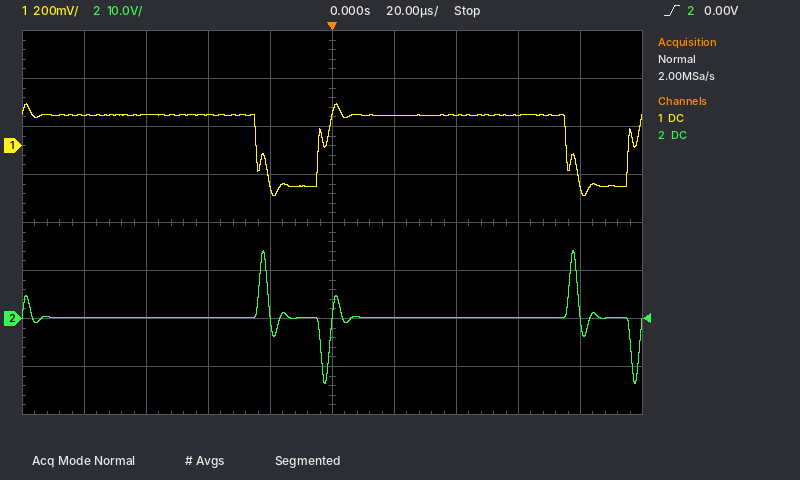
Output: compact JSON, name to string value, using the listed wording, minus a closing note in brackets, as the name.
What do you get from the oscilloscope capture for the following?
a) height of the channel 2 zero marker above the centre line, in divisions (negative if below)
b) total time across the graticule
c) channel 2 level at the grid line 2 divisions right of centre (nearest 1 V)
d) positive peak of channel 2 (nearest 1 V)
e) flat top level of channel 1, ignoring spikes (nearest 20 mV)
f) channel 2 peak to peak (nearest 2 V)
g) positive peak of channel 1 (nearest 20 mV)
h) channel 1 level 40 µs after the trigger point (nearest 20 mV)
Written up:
{"height of the channel 2 zero marker above the centre line, in divisions": "-2.0 div", "total time across the graticule": "200 µs", "channel 2 level at the grid line 2 divisions right of centre": "0 V", "positive peak of channel 2": "14 V", "flat top level of channel 1, ignoring spikes": "120 mV", "channel 2 peak to peak": "28 V", "positive peak of channel 1": "180 mV", "channel 1 level 40 µs after the trigger point": "120 mV"}
